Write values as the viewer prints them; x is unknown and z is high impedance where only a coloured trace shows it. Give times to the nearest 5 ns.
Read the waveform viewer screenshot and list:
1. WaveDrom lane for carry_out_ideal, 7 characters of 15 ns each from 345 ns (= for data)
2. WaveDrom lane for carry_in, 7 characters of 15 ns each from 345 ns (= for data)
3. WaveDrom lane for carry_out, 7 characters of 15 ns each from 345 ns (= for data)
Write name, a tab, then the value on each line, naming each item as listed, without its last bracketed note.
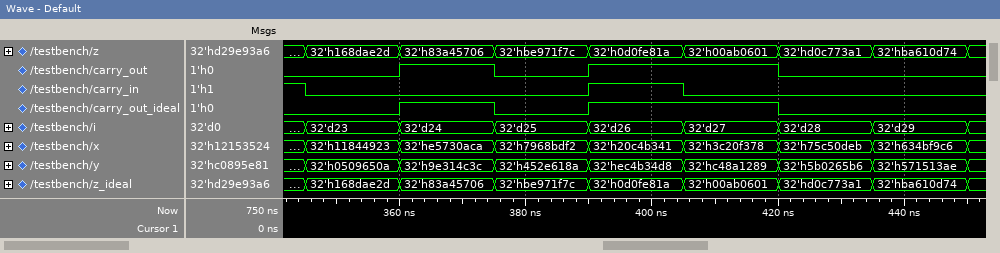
WaveDrom lane for carry_out_ideal, 7 characters of 15 ns each from 345 ns	{name: 'carry_out_ideal', wave: '0101.0.'}
WaveDrom lane for carry_in, 7 characters of 15 ns each from 345 ns	{name: 'carry_in', wave: '0..10..'}
WaveDrom lane for carry_out, 7 characters of 15 ns each from 345 ns	{name: 'carry_out', wave: '0101.0.'}
